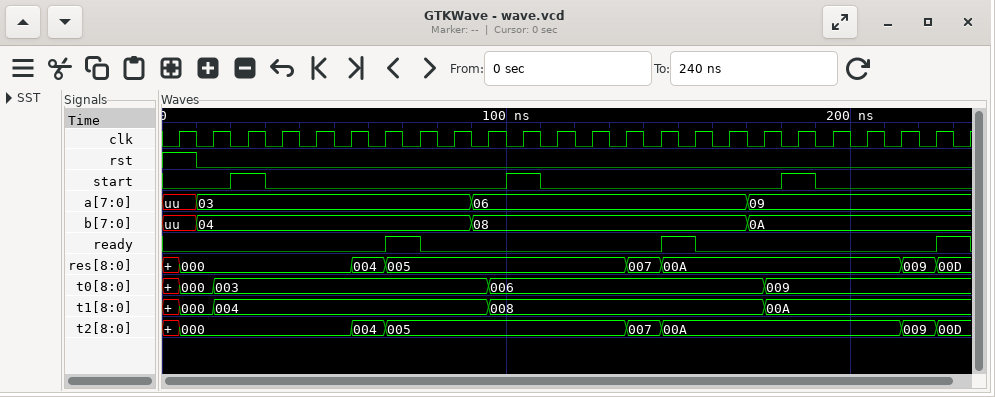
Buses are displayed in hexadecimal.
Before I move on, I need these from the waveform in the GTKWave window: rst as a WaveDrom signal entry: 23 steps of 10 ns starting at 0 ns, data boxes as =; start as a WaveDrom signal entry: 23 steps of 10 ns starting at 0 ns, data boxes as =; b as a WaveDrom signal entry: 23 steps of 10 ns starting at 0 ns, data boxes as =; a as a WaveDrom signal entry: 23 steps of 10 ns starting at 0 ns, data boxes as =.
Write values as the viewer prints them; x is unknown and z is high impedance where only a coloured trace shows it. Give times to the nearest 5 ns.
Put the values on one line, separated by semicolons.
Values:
{name: 'rst', wave: '10.....................'}; {name: 'start', wave: '0.10......10......10...'}; {name: 'b', wave: 'x=.......=.......=.....', data: '04 08 0A'}; {name: 'a', wave: 'x=.......=.......=.....', data: '03 06 09'}
